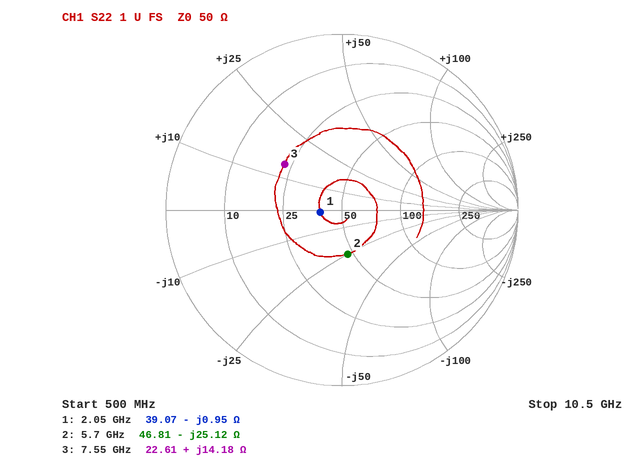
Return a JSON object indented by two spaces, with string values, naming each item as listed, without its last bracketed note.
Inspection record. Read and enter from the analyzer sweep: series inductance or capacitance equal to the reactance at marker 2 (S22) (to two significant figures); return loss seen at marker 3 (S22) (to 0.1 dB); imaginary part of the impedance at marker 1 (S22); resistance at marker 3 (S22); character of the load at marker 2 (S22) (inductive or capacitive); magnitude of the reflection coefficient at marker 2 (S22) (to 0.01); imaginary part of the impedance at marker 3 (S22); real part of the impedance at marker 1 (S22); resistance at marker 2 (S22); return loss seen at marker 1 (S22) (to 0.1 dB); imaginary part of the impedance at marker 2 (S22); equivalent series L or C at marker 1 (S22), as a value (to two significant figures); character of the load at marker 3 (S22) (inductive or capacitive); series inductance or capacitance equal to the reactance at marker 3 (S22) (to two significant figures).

{
  "series inductance or capacitance equal to the reactance at marker 2 (S22)": "1.1 pF",
  "return loss seen at marker 3 (S22)": "7.6 dB",
  "imaginary part of the impedance at marker 1": "-0.95 Ω",
  "resistance at marker 3": "22.61 Ω",
  "character of the load at marker 2 (S22)": "capacitive",
  "magnitude of the reflection coefficient at marker 2 (S22)": "0.25",
  "imaginary part of the impedance at marker 3": "+14.18 Ω",
  "real part of the impedance at marker 1": "39.07 Ω",
  "resistance at marker 2": "46.81 Ω",
  "return loss seen at marker 1 (S22)": "18.2 dB",
  "imaginary part of the impedance at marker 2": "-25.12 Ω",
  "equivalent series L or C at marker 1 (S22), as a value": "82 pF",
  "character of the load at marker 3 (S22)": "inductive",
  "series inductance or capacitance equal to the reactance at marker 3 (S22)": "300 pH"
}
